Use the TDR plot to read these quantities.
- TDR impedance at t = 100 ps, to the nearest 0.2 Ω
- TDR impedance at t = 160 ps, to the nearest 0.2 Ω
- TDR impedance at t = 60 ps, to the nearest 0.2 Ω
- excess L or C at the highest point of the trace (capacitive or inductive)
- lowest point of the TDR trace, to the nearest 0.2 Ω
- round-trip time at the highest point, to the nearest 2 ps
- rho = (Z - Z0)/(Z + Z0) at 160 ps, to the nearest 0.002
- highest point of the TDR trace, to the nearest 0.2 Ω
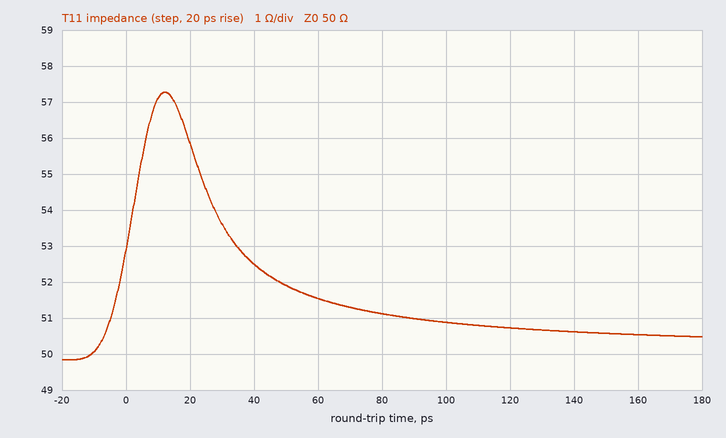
50.8 Ω
50.6 Ω
51.6 Ω
inductive
49.8 Ω
12 ps
+0.006
57.2 Ω
